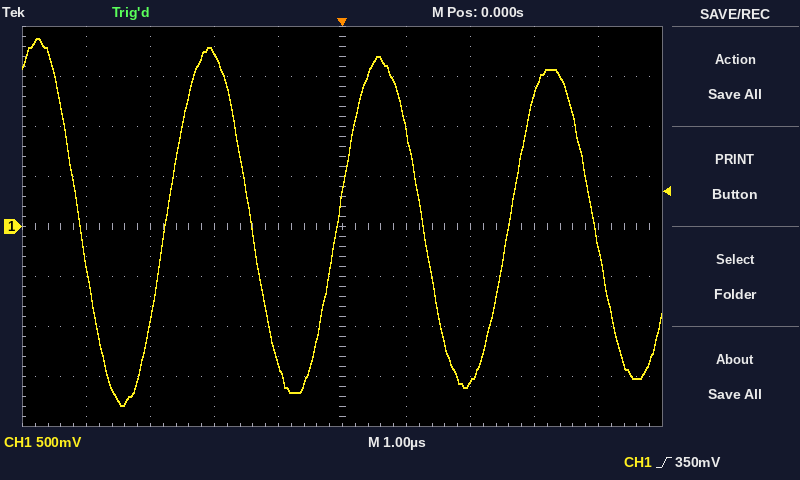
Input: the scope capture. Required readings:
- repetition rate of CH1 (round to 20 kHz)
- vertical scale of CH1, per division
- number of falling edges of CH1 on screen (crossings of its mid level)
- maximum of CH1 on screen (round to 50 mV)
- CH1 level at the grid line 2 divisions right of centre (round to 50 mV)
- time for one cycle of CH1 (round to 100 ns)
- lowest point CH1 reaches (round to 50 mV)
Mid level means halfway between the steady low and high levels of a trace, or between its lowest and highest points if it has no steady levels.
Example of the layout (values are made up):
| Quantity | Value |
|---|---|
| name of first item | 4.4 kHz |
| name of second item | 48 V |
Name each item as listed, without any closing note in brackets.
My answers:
| Quantity | Value |
|---|---|
| repetition rate of CH1 | 380 kHz |
| vertical scale of CH1, per division | 500 mV |
| number of falling edges of CH1 on screen | 4 |
| maximum of CH1 on screen | 1.90 V |
| CH1 level at the grid line 2 divisions right of centre | -1.55 V |
| time for one cycle of CH1 | 2.7 µs |
| lowest point CH1 reaches | -1.80 V |
